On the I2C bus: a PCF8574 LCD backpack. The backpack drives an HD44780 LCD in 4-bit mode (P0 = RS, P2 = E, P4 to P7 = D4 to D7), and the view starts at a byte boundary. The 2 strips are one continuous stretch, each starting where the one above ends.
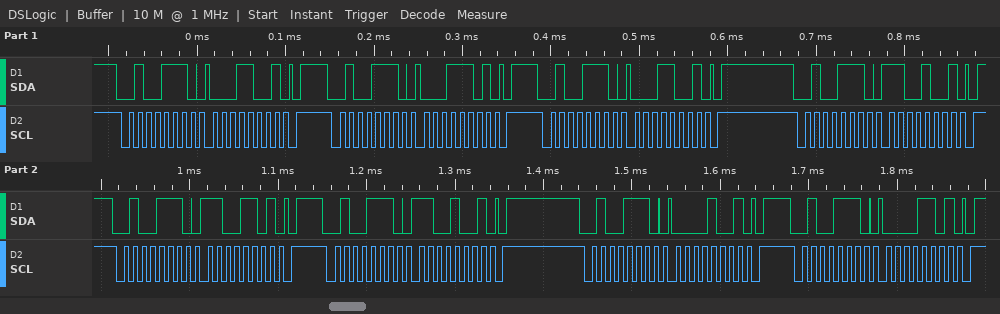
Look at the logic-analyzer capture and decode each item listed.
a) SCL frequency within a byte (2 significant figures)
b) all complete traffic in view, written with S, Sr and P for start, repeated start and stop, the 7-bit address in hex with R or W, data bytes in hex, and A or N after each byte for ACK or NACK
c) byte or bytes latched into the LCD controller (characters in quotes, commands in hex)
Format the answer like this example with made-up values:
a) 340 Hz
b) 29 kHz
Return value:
a) 100 kHz
b) S 27W A 19 A P S 27W A 1D A P S 27W A 19 A P S 27W A C9 A P S 27W A CD A P S 27W A C9 A P S 27W A 09 A P S 27W A 0D A P
c) data 0x1C
